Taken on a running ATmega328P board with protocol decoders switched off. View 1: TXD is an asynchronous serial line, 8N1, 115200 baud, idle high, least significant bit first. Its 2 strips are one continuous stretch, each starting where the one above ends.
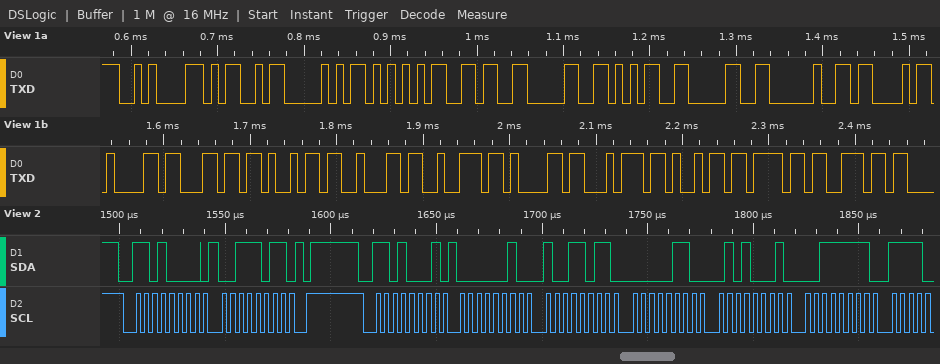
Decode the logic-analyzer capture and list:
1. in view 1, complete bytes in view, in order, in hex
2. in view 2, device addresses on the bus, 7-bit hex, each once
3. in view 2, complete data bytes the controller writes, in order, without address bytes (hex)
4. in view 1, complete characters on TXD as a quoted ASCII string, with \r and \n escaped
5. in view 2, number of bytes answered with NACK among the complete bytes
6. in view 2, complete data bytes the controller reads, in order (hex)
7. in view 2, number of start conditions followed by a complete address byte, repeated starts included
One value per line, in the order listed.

0x0A 0x4D 0x50 0x55 0x36 0x30 0x35 0x30 0x20 0x43 0x61 0x6C 0x69 0x62 0x72 0x61 0x74 0x69 0x6F 0x6E
0x68
3B
"\nMPU6050 Calibration"
0
02 9B 06 51 3F
2
